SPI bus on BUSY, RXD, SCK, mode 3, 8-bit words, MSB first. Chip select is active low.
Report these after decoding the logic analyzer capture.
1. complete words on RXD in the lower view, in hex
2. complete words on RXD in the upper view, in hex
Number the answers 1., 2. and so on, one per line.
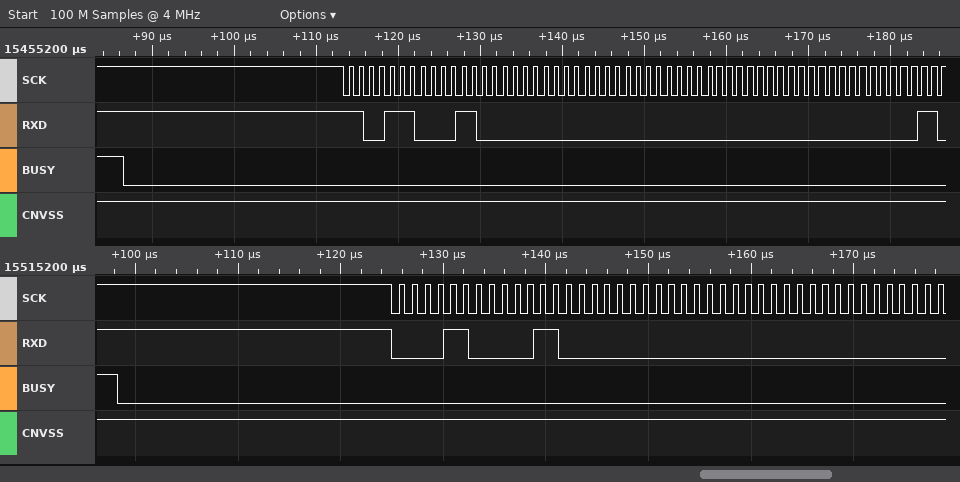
1. 0C, 18, 00, 00, 00
2. CE, 18, 00, 00, 00, 00, 00
